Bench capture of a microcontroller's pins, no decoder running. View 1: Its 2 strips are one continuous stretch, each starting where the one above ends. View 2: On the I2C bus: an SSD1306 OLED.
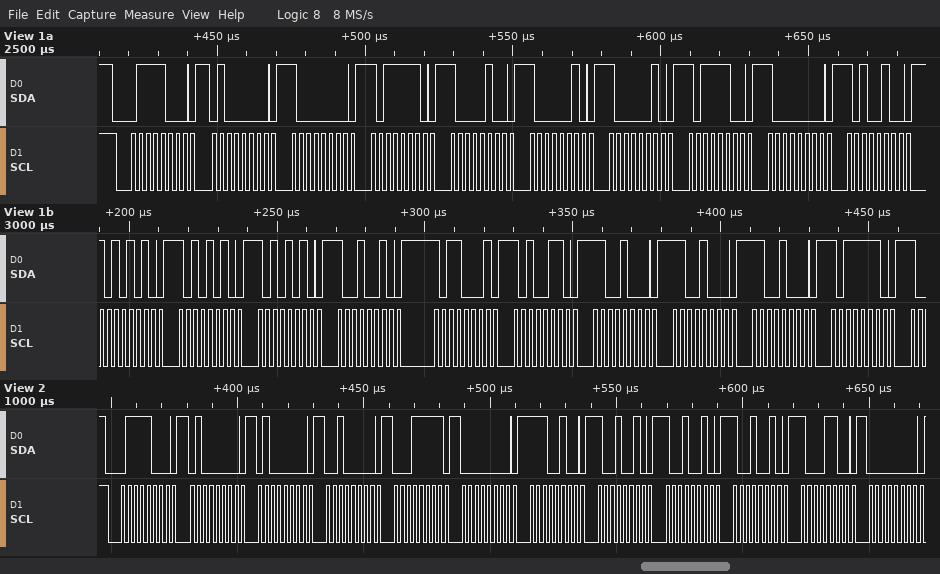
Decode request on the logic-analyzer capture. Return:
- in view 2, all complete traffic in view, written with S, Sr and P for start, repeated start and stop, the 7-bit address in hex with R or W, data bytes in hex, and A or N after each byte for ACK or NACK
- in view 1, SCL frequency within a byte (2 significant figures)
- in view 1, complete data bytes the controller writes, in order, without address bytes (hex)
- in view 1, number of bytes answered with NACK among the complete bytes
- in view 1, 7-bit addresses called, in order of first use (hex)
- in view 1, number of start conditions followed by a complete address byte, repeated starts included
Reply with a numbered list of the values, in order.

1. S 3CW A 40 A 40 A 20 A 1F A 00 A E4 A 92 A 92 A 92 A 8C A 00 A
2. 400 kHz
3. 40 80 BE 84 82 82 BC 80 A4 AA AA AA 92 B1 A6 C8 C8 C8 BE
4. 0
5. 0x3C
6. 1
